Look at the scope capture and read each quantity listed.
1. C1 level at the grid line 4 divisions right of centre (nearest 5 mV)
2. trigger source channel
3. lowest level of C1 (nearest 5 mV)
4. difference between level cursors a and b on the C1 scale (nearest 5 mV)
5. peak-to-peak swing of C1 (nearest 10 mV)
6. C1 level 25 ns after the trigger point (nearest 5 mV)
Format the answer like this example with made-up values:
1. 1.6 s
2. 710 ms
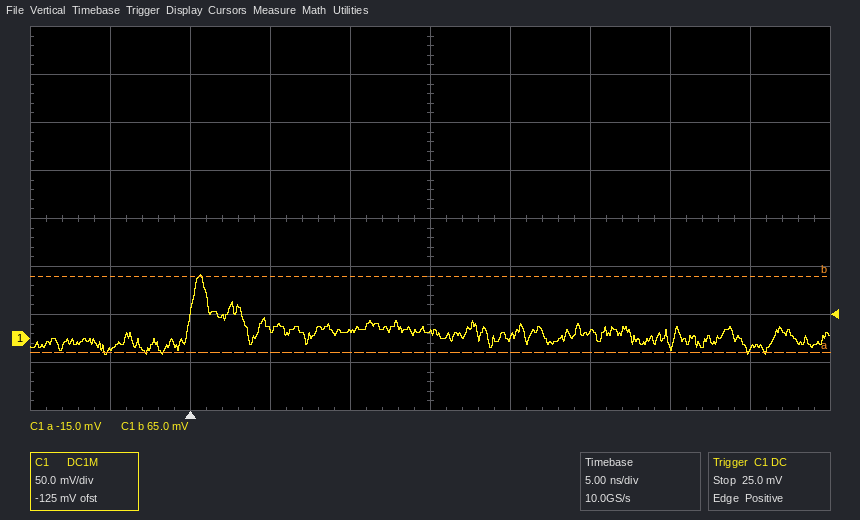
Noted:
1. -10 mV
2. C1
3. -15 mV
4. 80 mV
5. 80 mV
6. 5 mV
